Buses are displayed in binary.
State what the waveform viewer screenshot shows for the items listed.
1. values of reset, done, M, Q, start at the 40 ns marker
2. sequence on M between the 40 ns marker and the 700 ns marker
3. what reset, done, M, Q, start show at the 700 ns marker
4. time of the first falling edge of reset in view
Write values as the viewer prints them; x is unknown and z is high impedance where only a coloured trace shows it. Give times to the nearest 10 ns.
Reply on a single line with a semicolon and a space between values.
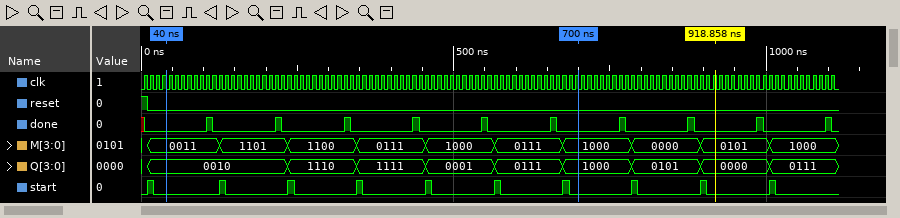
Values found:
reset=0, done=0, M=0011, Q=0010, start=0; 0011, 1101, 1100, 0111, 1000, 0111, 1000; reset=0, done=0, M=1000, Q=1000, start=0; 10 ns
